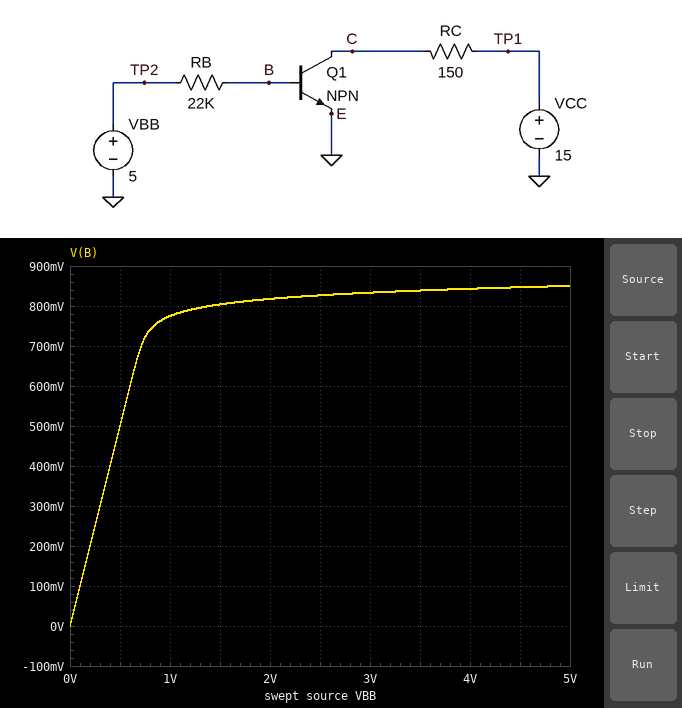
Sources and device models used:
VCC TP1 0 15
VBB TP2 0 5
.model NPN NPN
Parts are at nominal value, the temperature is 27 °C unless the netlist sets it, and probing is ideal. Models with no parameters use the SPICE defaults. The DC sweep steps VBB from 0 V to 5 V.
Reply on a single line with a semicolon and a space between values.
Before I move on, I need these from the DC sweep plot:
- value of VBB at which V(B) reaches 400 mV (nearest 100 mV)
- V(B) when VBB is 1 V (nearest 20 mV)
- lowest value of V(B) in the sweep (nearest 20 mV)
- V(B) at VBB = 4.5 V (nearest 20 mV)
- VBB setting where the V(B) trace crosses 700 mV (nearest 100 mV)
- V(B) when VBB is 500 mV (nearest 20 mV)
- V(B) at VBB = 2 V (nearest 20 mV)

400 mV; 780 mV; 0 V; 840 mV; 700 mV; 500 mV; 820 mV
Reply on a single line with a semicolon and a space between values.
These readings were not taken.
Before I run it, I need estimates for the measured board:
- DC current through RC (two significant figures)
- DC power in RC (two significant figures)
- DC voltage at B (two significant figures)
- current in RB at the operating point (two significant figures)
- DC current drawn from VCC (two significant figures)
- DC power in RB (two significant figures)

19 mA; 53 mW; 850 mV; 190 µA; 19 mA; 780 µW
